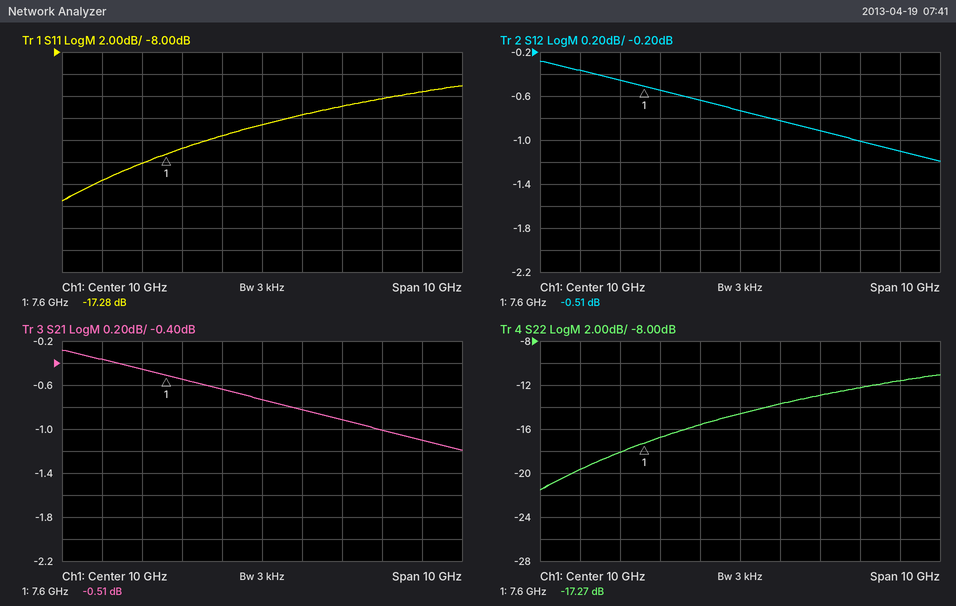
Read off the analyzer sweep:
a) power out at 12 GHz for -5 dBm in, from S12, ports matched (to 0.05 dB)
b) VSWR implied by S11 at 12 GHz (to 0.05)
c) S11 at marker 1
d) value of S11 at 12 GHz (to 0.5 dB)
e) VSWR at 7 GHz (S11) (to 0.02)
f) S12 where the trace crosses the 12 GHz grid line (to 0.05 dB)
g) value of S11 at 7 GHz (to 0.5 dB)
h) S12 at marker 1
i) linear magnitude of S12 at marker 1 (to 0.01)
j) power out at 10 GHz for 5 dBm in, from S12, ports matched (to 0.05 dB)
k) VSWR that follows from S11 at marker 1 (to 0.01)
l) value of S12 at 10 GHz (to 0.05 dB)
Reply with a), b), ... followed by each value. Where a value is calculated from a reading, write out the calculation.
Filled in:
a) -5 dBm + (-0.90 dB) = -5.90 dBm
b) |Γ| = 10^(-13/20) = 0.2239; VSWR = (1 + 0.2239)/(1 − 0.2239) ≈ 1.58, so 1.60 to the nearest 0.05
c) -17.28 dB
d) -13.0 dB
e) |Γ| = 10^(-18/20) = 0.1259; VSWR = (1 + 0.1259)/(1 − 0.1259) ≈ 1.29, so 1.28 to the nearest 0.02
f) -0.90 dB
g) -18.0 dB
h) -0.51 dB
i) 10^(-0.51/20) ≈ 0.94
j) 5 dBm + (-0.75 dB) = 4.25 dBm
k) (1 + 0.1368)/(1 − 0.1368) ≈ 1.32
l) -0.75 dB
